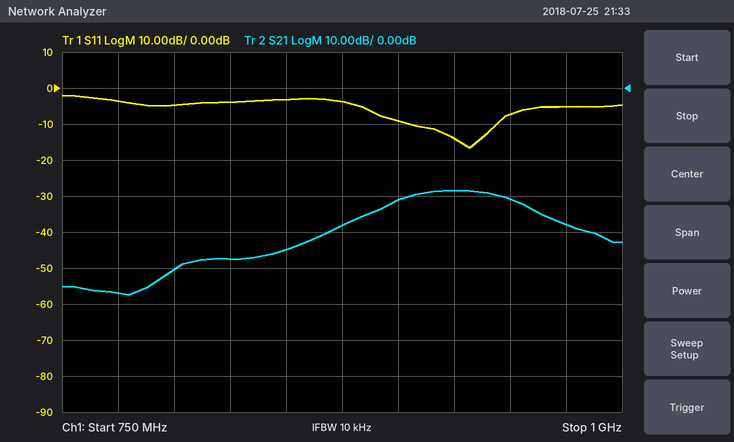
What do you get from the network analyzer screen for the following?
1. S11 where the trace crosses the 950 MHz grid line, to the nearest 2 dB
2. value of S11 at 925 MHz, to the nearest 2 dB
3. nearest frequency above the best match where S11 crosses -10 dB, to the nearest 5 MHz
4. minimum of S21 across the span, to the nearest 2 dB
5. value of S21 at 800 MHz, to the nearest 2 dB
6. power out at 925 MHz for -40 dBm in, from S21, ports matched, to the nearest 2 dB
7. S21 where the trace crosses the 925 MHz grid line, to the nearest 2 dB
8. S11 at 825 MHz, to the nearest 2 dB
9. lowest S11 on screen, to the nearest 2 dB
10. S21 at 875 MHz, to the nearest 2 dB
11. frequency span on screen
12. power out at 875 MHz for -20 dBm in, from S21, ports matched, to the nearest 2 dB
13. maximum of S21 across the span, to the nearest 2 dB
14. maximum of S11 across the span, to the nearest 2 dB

-8 dB
-14 dB
945 MHz
-58 dB
-50 dB
-68 dBm
-28 dB
-4 dB
-16 dB
-38 dB
250 MHz
-58 dBm
-28 dB
-2 dB
